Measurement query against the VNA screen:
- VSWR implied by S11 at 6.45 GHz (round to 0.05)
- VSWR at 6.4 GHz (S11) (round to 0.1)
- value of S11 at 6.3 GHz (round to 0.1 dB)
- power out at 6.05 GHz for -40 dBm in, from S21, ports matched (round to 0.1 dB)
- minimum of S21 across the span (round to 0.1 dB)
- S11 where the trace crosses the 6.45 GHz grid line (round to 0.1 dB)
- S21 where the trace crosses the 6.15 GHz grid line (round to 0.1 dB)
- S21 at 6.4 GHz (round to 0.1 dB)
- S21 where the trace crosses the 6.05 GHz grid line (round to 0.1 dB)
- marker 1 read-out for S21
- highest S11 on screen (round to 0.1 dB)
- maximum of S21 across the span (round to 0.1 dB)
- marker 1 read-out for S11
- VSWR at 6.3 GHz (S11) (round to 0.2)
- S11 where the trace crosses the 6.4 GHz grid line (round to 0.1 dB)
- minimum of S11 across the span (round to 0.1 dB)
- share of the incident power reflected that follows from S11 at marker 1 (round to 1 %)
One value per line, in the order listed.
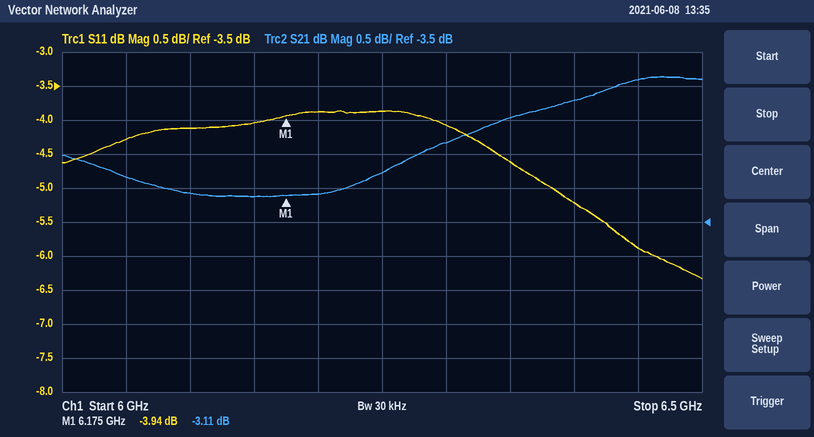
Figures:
3.05
3.4
-4.1 dB
-42.8 dBm
-3.1 dB
-5.9 dB
-3.1 dB
-1.7 dB
-2.8 dB
-3.11 dB
-3.9 dB
-1.4 dB
-3.94 dB
4.4
-5.2 dB
-6.3 dB
40 %
